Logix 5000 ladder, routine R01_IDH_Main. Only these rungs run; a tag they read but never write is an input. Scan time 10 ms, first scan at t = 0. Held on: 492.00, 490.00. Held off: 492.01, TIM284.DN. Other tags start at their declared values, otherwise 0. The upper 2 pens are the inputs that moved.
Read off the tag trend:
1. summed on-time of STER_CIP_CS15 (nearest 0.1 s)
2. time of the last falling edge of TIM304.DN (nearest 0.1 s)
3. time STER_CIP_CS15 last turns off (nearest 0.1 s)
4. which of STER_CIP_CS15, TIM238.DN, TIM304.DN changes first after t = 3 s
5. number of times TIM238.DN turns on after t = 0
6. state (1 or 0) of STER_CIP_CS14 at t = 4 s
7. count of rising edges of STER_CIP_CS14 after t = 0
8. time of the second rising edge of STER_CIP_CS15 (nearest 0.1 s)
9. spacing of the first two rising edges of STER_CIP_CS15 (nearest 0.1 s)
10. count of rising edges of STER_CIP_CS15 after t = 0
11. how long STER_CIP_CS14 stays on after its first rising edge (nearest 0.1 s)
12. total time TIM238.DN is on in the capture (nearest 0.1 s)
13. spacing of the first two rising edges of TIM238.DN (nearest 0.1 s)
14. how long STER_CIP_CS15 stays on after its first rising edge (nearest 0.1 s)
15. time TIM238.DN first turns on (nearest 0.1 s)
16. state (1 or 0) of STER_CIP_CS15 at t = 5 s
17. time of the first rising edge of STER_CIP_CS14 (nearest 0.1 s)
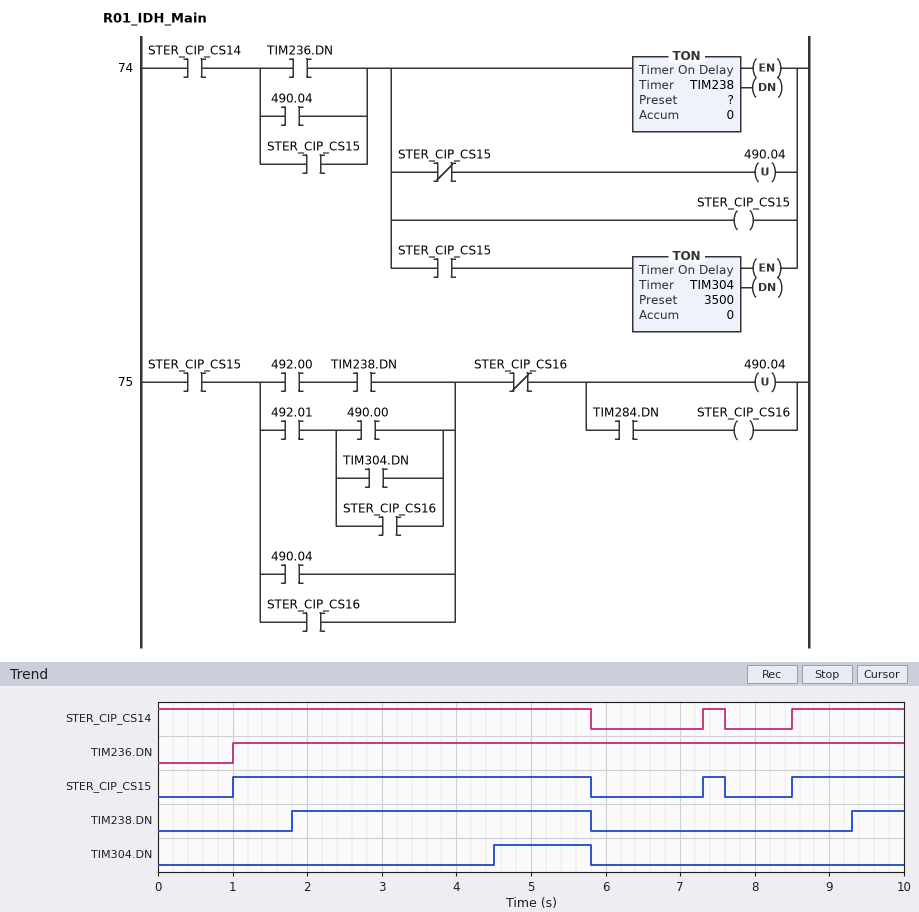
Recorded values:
6.6 s
5.8 s
7.6 s
TIM304.DN
2
1
2
7.3 s
6.3 s
3
0.3 s
4.7 s
7.5 s
4.8 s
1.8 s
1
7.3 s
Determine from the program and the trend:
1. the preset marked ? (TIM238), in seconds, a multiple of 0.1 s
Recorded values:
0.8 s
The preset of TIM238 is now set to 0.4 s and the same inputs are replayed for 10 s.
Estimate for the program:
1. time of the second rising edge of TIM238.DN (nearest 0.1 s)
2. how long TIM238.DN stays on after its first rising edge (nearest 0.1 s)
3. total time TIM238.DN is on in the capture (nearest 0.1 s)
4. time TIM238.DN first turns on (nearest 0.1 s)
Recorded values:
8.9 s
4.4 s
5.5 s
1.4 s
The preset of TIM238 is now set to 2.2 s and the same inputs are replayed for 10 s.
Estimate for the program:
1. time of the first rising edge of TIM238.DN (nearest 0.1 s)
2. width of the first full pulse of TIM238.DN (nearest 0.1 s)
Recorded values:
3.2 s
2.6 s
